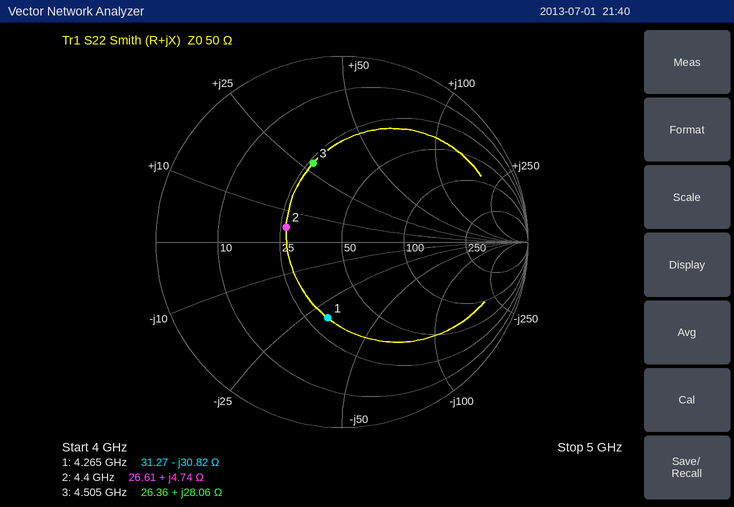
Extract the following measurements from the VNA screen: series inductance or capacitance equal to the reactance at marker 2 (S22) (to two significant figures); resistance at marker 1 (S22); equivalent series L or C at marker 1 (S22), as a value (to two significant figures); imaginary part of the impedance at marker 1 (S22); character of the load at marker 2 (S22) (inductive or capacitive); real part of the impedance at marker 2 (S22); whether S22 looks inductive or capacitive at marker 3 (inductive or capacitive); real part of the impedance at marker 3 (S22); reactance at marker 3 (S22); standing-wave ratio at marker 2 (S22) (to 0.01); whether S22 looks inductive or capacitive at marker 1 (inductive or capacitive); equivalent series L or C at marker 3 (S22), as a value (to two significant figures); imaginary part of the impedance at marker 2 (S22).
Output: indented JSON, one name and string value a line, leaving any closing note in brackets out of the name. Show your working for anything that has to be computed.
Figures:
{
  "series inductance or capacitance equal to the reactance at marker 2 (S22)": "L = 4.74 Ω/(2π × 4.4 GHz) ≈ 171 pH, so 170 pH to two significant figures",
  "resistance at marker 1": "31.27 Ω",
  "equivalent series L or C at marker 1 (S22), as a value": "C = 1/(2π × 4.265 GHz × 30.82 Ω) ≈ 1.2 pF",
  "imaginary part of the impedance at marker 1": "-30.82 Ω",
  "character of the load at marker 2 (S22)": "inductive",
  "real part of the impedance at marker 2": "26.61 Ω",
  "whether S22 looks inductive or capacitive at marker 3": "inductive",
  "real part of the impedance at marker 3": "26.36 Ω",
  "reactance at marker 3": "+28.06 Ω",
  "standing-wave ratio at marker 2 (S22)": "1.90",
  "whether S22 looks inductive or capacitive at marker 1": "capacitive",
  "equivalent series L or C at marker 3 (S22), as a value": "L = 28.06 Ω/(2π × 4.505 GHz) ≈ 991 pH, so 990 pH to two significant figures",
  "imaginary part of the impedance at marker 2": "+4.74 Ω"
}
